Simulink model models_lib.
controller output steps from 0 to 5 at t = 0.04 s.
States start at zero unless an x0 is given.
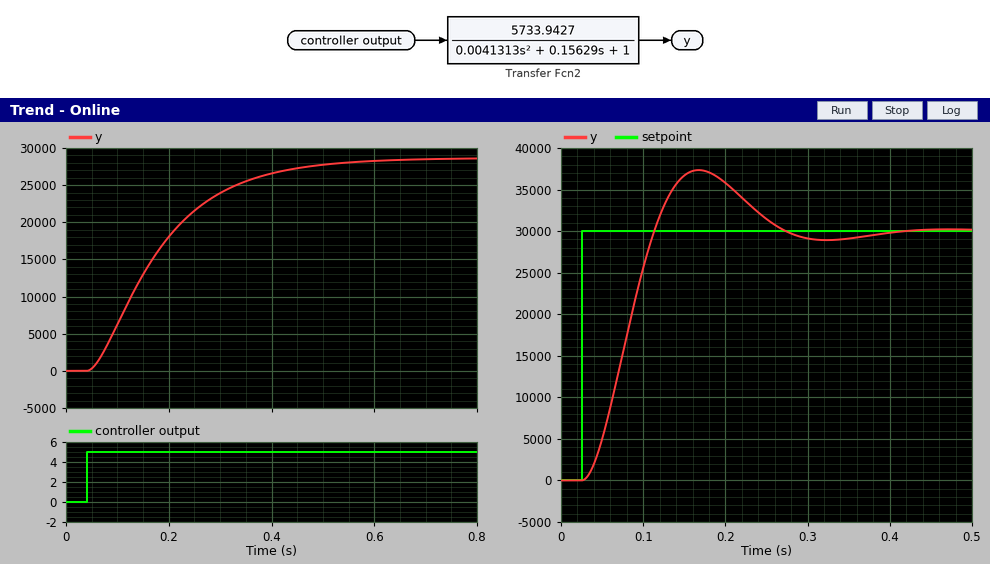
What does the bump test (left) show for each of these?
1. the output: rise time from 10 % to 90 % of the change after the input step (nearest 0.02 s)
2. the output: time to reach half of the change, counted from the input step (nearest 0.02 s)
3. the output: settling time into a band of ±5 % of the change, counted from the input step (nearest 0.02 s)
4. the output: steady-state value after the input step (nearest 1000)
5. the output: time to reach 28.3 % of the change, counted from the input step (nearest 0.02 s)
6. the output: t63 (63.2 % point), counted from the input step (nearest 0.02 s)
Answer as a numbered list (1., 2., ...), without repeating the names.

1. 0.28 s
2. 0.12 s
3. 0.40 s
4. 29000
5. 0.08 s
6. 0.16 s
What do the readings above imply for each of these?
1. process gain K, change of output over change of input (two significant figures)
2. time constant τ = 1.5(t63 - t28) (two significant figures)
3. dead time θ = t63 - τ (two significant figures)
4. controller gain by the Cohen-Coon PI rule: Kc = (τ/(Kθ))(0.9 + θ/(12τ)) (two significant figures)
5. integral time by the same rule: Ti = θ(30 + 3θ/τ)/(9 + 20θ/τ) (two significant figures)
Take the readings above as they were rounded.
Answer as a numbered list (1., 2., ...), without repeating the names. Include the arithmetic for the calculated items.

1. (29000 - 0) / 5 = 5800
2. 1.5 × (0.16 - 0.08) = 0.12 s
3. 0.16 - 0.12 = 0.040 s
4. 0.12 / (5800 × 0.04) × (0.9 + 0.04 / (12 × 0.12)) = 0.00048
5. 0.04 × (30 + 3 × 0.04 / 0.12) / (9 + 20 × 0.04 / 0.12) = 0.079 s
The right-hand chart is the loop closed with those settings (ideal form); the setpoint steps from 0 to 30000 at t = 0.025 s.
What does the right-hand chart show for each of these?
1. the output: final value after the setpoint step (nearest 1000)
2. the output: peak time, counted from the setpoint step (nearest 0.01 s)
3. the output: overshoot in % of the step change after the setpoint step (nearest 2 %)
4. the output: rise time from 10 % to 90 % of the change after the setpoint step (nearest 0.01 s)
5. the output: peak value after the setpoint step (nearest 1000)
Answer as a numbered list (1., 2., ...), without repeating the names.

1. 30000
2. 0.14 s
3. 24 %
4. 0.06 s
5. 37000
